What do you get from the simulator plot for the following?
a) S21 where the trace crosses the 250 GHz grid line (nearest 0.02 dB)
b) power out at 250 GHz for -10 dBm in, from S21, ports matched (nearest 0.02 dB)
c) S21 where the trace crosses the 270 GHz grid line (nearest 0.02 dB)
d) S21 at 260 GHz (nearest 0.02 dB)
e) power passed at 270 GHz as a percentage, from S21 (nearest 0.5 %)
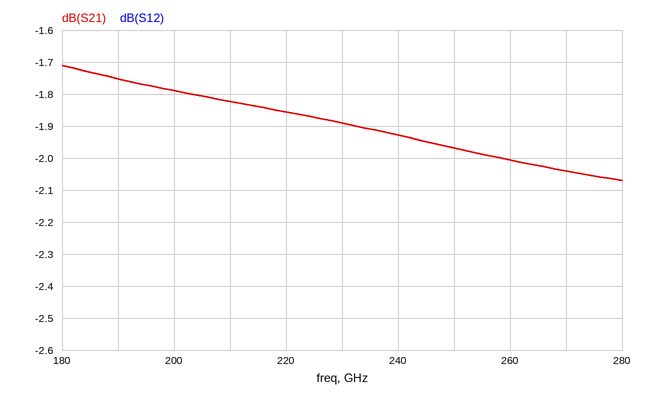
-1.96 dB
-11.96 dBm
-2.04 dB
-2.00 dB
62.5 %
